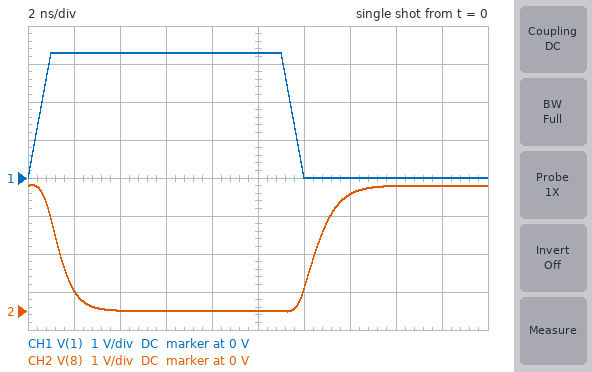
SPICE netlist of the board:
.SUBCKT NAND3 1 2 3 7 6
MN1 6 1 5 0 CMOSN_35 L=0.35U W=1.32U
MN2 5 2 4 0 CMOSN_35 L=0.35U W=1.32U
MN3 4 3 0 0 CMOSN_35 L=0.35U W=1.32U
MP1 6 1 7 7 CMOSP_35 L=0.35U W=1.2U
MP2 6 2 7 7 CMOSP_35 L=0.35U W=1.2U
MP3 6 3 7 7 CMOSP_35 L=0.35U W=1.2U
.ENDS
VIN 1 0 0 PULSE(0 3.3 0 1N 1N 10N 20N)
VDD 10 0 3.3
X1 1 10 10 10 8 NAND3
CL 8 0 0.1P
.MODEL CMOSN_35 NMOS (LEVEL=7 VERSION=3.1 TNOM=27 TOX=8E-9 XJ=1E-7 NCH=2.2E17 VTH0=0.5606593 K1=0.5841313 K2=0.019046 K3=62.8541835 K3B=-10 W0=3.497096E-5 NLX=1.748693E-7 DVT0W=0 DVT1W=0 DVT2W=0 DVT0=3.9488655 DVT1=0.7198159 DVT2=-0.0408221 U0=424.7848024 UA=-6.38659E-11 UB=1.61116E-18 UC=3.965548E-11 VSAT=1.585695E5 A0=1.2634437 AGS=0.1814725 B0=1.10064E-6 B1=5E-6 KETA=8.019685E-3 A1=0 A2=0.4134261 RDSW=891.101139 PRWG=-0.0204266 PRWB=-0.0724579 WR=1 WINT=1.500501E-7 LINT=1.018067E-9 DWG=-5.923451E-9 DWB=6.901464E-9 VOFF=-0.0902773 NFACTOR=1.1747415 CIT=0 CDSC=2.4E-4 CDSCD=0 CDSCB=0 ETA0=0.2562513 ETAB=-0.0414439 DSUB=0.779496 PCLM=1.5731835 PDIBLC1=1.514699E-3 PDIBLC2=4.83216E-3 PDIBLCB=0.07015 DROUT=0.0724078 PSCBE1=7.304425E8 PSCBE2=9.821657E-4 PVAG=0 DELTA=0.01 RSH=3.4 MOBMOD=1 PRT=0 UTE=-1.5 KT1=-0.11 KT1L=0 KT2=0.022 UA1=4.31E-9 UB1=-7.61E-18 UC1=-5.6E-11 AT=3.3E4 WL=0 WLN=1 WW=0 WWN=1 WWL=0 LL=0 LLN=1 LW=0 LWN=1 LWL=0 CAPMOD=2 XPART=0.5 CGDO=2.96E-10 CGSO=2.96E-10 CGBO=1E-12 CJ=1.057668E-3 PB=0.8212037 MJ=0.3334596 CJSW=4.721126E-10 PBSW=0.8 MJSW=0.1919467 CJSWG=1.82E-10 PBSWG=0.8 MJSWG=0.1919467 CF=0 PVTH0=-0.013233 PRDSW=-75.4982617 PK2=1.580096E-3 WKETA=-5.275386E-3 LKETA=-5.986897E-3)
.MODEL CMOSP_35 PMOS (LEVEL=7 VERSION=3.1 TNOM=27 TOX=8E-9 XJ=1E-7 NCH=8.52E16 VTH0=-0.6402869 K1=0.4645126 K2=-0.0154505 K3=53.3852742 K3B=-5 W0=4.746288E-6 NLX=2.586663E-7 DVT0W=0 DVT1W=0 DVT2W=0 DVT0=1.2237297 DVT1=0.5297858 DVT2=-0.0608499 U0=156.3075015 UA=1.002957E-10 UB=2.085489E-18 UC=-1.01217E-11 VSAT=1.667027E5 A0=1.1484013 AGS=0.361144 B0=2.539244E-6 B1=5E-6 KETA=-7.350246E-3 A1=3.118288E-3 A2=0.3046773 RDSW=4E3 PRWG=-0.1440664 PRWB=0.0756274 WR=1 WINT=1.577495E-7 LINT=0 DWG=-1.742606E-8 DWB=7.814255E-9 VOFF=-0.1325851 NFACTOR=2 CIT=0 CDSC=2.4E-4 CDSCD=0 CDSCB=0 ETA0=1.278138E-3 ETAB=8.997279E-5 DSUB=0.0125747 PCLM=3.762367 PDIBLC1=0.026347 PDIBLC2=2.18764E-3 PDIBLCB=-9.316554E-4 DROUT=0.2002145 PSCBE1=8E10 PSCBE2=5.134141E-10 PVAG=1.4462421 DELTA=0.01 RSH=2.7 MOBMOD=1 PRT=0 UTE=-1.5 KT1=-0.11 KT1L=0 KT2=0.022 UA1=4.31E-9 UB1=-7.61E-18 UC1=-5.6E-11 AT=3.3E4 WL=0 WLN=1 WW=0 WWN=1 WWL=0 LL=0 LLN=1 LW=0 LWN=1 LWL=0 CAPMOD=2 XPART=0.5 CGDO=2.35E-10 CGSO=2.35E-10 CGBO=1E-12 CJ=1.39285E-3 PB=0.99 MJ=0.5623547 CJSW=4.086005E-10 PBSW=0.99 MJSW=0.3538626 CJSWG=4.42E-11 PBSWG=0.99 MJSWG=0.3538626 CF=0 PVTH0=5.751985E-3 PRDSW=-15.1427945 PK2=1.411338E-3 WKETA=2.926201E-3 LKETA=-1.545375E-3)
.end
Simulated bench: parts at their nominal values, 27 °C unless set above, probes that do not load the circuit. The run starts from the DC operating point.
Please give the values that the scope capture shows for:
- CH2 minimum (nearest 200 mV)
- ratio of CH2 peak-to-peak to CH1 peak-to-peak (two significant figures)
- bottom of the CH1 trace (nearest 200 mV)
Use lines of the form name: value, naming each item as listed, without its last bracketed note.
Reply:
CH2 minimum: 0 V
ratio of CH2 peak-to-peak to CH1 peak-to-peak: 1.0
bottom of the CH1 trace: 0 V
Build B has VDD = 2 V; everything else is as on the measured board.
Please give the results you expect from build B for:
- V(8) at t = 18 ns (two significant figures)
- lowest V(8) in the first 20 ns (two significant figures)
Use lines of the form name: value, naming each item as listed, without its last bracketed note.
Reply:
V(8) at t = 18 ns: 2.0 V
lowest V(8) in the first 20 ns: -28 mV
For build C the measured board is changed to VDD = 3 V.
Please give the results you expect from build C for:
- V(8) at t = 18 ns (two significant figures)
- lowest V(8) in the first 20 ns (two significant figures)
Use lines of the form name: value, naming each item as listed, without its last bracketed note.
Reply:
V(8) at t = 18 ns: 3.0 V
lowest V(8) in the first 20 ns: -17 mV
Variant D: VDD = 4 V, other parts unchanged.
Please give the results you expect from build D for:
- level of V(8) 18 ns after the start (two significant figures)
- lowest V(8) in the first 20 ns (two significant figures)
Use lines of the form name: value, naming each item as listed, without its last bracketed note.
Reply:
level of V(8) 18 ns after the start: 4.0 V
lowest V(8) in the first 20 ns: -3.0 mV
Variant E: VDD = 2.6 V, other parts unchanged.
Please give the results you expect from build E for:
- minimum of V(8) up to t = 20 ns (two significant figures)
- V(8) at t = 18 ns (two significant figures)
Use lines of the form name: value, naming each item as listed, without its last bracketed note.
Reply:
minimum of V(8) up to t = 20 ns: -21 mV
V(8) at t = 18 ns: 2.6 V
